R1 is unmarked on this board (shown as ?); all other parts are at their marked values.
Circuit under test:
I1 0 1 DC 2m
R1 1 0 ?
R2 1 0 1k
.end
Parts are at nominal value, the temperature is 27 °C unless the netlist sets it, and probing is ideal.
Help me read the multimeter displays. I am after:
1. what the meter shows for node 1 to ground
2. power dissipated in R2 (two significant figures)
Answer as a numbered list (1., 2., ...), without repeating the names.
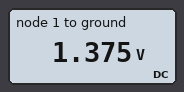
1. 1.375 V
2. 1.9 mW
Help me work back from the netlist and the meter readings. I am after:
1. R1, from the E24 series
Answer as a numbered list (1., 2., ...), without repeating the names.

1. 2.2 kΩ
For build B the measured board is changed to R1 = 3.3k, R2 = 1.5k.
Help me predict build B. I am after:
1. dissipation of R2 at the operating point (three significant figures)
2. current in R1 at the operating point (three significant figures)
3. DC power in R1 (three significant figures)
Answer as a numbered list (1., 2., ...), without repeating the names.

1. 2.84 mW
2. 625 µA
3. 1.29 mW
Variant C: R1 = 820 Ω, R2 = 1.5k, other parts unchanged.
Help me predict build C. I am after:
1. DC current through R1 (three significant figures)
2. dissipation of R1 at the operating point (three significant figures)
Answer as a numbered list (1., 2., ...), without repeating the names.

1. 1.29 mA
2. 1.37 mW
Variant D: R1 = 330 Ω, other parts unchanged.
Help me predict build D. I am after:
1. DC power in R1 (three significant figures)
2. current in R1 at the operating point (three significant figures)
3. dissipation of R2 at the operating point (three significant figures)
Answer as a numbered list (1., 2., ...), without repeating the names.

1. 746 µW
2. 1.50 mA
3. 246 µW
